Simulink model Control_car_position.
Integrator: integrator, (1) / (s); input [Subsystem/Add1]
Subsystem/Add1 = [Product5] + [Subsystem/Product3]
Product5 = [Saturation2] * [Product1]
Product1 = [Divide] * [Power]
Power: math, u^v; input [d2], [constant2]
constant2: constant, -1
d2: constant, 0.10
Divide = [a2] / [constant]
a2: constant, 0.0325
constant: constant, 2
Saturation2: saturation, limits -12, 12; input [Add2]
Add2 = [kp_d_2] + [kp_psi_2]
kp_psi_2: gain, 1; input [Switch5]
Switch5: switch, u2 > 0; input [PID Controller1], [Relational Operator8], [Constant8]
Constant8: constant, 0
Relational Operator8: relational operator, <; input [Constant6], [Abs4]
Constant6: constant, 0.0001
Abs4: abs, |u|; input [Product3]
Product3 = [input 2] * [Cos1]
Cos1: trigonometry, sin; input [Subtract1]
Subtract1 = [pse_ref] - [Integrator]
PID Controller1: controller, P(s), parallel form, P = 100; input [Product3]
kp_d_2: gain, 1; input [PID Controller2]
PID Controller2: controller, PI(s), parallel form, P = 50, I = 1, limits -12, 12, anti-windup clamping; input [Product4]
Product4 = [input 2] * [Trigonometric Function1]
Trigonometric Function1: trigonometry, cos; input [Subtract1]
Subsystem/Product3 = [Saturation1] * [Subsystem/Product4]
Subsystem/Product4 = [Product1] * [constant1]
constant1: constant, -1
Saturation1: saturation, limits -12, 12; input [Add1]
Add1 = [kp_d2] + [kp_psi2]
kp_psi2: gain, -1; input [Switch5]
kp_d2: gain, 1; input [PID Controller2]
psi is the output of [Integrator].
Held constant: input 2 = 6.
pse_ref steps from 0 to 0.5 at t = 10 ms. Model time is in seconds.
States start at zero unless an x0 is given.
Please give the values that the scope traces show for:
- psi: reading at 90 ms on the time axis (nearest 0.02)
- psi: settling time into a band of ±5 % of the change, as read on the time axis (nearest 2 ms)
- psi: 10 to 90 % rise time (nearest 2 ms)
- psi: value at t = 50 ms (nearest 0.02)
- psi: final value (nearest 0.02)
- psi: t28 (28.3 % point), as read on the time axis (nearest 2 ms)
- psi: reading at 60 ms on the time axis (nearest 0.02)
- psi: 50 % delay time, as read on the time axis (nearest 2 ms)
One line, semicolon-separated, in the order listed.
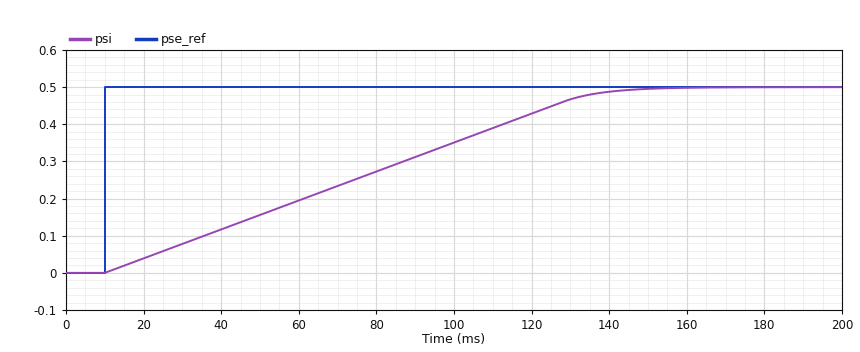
0.32; 132 ms; 102 ms; 0.16; 0.50; 46 ms; 0.20; 74 ms
